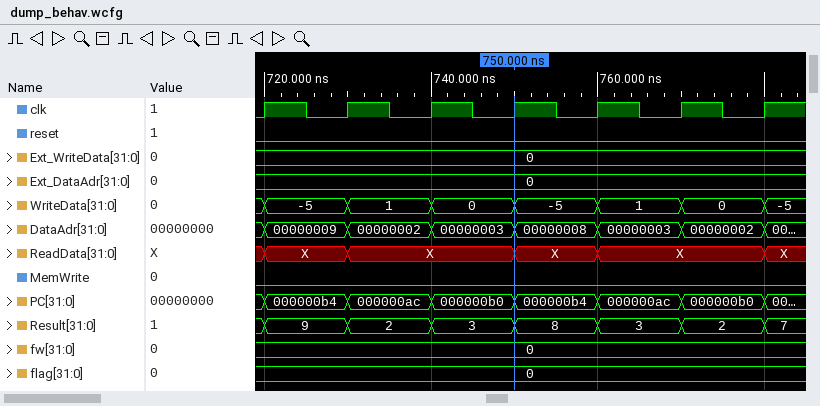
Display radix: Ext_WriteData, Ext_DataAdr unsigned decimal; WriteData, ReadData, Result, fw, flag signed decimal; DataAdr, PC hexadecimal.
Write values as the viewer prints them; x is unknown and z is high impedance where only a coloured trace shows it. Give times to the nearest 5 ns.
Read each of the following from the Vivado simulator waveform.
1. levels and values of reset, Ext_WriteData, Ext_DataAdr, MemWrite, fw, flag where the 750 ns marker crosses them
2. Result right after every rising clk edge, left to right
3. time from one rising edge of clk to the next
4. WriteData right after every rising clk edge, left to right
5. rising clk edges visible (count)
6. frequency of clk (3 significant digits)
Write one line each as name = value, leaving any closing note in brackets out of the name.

levels and values of reset, Ext_WriteData, Ext_DataAdr, MemWrite, fw, flag where the 750 ns marker crosses them = reset=0, Ext_WriteData=0, Ext_DataAdr=0, MemWrite=0, fw=0, flag=0
Result right after every rising clk edge, left to right = 9, 2, 3, 8, 3, 2, 7
time from one rising edge of clk to the next = 10 ns
WriteData right after every rising clk edge, left to right = -5, 1, 0, -5, 1, 0, -5
rising clk edges visible = 7
frequency of clk = 100 MHz
